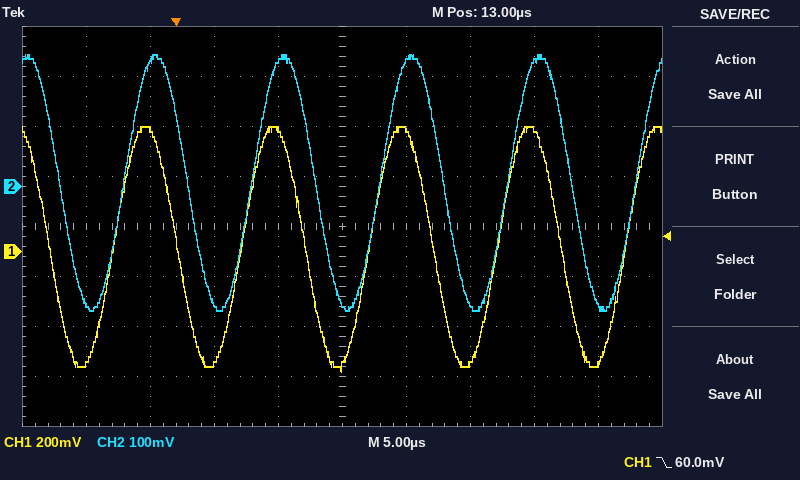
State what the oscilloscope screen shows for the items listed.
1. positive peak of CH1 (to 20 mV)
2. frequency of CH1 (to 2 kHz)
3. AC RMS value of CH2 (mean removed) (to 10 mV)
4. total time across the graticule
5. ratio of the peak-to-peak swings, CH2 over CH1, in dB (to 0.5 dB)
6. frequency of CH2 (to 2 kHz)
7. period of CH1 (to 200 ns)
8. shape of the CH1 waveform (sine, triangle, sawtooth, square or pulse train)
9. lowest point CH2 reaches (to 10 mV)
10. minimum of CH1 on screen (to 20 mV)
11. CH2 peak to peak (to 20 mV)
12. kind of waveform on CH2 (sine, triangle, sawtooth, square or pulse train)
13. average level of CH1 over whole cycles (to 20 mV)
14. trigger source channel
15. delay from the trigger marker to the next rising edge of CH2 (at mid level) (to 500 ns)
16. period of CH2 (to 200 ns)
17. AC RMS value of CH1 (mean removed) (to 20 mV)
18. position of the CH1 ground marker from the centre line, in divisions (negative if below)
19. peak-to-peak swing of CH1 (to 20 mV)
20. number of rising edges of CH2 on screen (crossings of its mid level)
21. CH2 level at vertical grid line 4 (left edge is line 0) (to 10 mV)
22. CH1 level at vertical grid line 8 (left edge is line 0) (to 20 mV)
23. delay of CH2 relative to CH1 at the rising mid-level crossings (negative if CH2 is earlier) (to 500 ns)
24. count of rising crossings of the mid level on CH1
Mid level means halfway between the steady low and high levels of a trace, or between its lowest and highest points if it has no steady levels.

500 mV
100 kHz
180 mV
50 µs
-5.5 dB
100 kHz
10.0 µs
sine
-250 mV
-480 mV
520 mV
sine
20 mV
CH1
6.0 µs
10.0 µs
340 mV
-0.5 div
980 mV
5
250 mV
480 mV
+1.0 µs
5
